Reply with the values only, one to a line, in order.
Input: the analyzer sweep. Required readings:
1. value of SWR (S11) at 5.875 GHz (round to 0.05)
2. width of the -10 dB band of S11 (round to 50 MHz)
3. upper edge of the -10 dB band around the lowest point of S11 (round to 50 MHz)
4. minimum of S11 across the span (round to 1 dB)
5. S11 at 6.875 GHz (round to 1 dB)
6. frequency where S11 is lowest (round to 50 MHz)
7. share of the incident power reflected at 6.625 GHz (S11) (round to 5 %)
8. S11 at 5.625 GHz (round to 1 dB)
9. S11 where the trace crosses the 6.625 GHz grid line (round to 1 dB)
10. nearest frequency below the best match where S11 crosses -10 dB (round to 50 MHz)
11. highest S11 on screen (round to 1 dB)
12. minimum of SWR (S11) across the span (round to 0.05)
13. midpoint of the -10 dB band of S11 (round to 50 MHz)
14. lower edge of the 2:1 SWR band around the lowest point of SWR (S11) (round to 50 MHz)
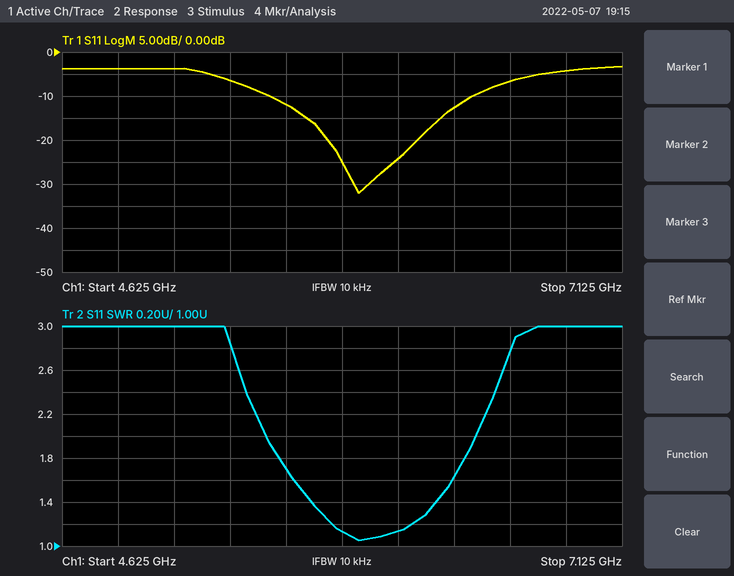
1.15
900 MHz
6.45 GHz
-32 dB
-4 dB
5.95 GHz
20 %
-12 dB
-7 dB
5.55 GHz
-3 dB
1.05
6.00 GHz
5.55 GHz
